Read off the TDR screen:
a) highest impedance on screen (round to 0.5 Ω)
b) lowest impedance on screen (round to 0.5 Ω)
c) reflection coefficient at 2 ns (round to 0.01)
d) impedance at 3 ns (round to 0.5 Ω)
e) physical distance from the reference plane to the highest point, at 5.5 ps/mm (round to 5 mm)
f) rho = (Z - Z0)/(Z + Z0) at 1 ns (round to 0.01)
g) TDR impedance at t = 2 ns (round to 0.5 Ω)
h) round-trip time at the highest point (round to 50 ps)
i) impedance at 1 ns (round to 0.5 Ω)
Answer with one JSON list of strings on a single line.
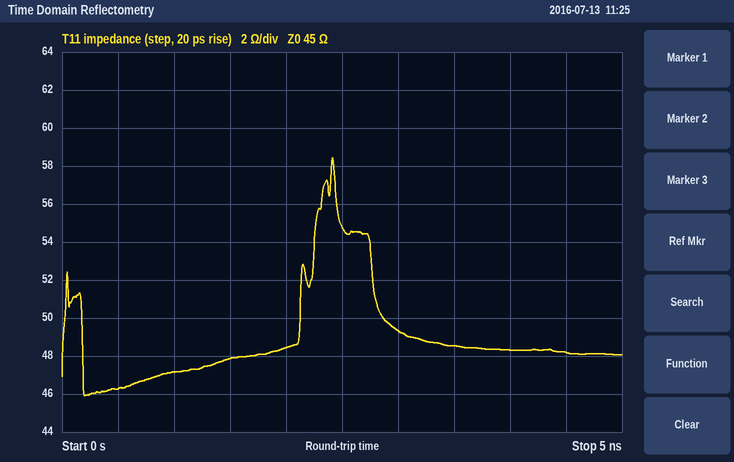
["58.5 Ω", "46.0 Ω", "+0.04", "49.5 Ω", "220 mm", "+0.02", "48.5 Ω", "2.40 ns", "47.0 Ω"]
